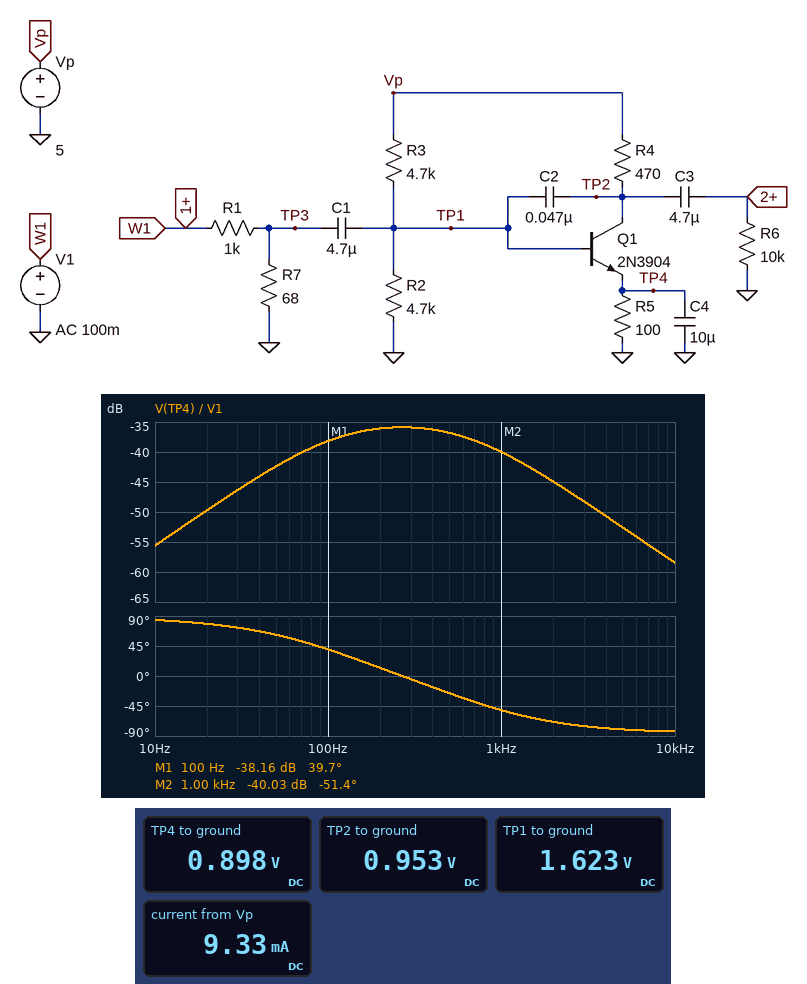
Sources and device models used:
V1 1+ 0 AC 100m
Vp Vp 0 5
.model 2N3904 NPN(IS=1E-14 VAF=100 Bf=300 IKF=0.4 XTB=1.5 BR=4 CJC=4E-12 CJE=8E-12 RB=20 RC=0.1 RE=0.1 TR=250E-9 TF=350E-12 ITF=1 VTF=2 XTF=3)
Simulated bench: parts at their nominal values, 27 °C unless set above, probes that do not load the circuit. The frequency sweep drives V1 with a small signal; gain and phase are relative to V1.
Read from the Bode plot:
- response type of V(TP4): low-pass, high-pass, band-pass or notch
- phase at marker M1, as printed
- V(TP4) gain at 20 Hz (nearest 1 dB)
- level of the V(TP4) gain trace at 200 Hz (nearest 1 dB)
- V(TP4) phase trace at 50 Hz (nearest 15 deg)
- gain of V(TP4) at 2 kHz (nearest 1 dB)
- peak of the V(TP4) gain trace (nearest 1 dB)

band-pass
39.7 deg
-50 dB
-36 dB
60 deg
-45 dB
-36 dB
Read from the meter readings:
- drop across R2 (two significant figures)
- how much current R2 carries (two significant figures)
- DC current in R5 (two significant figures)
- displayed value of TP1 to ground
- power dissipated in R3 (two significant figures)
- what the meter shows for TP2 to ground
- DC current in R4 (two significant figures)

1.6 V
350 µA
9.0 mA
1.623 V
2.4 mW
0.953 V
8.6 mA
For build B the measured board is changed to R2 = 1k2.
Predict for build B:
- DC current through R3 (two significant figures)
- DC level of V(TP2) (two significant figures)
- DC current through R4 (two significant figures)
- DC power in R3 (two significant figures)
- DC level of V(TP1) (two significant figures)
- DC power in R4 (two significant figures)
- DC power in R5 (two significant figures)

850 µA
3.5 V
3.2 mA
3.4 mW
1.0 V
4.8 mW
1.0 mW
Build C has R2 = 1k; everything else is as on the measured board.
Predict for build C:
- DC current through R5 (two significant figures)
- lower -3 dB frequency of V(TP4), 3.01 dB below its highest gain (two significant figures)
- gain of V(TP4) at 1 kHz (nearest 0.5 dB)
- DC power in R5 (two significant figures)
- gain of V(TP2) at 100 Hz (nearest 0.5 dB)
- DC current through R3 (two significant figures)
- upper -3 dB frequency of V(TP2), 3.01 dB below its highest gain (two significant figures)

2.0 mA
36 Hz
-28.0 dB
400 µW
-12.0 dB
880 µA
2.8 kHz
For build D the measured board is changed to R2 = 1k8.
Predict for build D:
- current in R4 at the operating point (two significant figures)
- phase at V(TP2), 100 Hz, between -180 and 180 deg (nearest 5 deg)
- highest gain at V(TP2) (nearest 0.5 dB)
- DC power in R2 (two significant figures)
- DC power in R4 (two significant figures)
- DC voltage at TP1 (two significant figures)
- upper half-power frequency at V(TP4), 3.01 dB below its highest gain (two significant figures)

6.5 mA
-140 deg
7.0 dB
1.0 mW
20 mW
1.4 V
1.7 kHz
